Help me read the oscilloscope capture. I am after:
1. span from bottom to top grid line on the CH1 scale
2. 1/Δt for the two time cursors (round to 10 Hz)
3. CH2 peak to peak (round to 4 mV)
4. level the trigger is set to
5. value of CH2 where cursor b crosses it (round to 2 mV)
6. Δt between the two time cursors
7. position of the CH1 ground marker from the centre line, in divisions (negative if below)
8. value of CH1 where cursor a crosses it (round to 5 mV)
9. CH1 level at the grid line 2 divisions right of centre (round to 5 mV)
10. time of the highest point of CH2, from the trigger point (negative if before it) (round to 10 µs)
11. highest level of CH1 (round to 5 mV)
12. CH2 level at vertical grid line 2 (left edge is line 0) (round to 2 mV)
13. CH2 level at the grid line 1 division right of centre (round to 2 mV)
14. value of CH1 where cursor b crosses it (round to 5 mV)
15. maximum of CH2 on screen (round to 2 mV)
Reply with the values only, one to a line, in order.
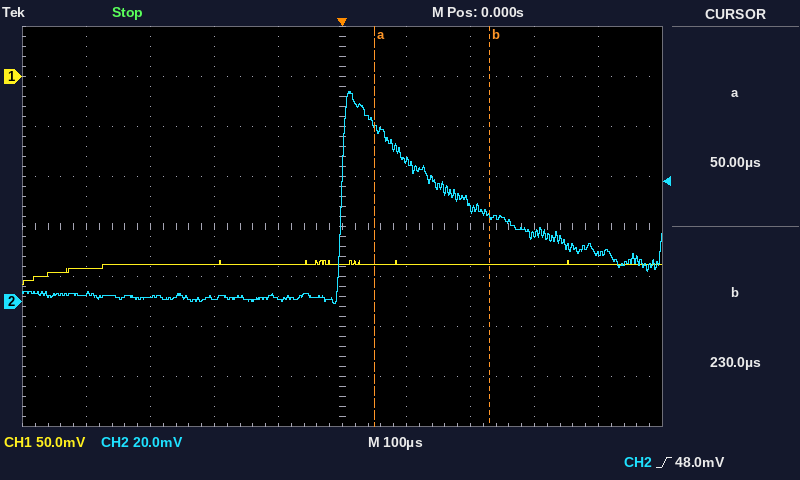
400 mV
5.56 kHz
84 mV
48.0 mV
34 mV
180 µs
+3.0 div
-190 mV
-190 mV
+10 µs
-185 mV
2 mV
56 mV
-190 mV
84 mV
